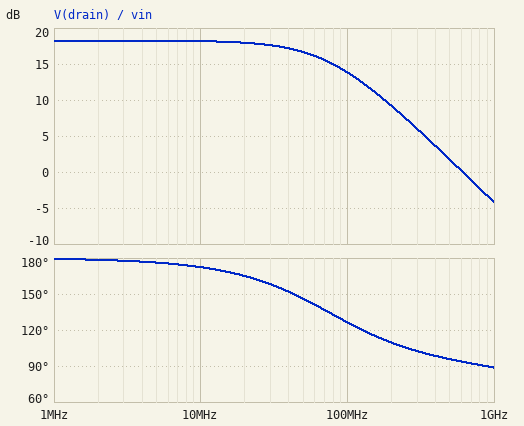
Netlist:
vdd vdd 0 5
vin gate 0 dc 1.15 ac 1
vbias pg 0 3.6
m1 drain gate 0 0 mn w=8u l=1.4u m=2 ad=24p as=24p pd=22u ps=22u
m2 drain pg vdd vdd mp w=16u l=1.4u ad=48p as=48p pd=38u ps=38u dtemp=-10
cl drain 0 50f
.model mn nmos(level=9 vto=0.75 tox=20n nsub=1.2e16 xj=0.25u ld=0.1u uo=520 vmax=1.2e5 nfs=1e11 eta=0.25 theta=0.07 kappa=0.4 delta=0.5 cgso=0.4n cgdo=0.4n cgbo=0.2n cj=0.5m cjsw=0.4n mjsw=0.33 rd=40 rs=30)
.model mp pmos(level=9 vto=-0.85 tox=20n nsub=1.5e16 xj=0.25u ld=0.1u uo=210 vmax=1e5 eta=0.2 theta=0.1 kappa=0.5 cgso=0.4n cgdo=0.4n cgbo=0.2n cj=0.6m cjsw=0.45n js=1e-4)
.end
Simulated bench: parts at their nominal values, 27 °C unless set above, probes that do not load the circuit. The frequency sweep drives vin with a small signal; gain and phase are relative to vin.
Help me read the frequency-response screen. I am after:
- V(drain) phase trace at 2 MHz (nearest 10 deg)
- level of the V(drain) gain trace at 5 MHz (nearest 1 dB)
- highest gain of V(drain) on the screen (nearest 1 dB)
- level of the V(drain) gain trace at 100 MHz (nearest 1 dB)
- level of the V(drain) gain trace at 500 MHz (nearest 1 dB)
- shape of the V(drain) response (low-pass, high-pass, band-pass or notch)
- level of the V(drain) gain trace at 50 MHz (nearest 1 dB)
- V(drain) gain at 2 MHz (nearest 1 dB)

180 deg
18 dB
18 dB
14 dB
2 dB
low-pass
17 dB
18 dB
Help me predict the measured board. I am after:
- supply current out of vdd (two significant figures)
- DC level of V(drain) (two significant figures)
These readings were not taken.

130 µA
1.2 V
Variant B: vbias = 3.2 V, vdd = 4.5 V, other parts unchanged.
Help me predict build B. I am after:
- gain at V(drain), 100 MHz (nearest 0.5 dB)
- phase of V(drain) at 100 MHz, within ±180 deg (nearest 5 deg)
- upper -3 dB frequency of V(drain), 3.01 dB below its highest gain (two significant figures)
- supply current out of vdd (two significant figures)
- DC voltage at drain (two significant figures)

13.0 dB
120 deg
64 MHz
100 µA
450 mV
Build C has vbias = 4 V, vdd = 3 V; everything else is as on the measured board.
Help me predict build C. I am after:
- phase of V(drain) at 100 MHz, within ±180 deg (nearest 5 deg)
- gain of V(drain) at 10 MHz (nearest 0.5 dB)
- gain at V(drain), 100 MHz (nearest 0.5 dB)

80 deg
-51.0 dB
-31.0 dB
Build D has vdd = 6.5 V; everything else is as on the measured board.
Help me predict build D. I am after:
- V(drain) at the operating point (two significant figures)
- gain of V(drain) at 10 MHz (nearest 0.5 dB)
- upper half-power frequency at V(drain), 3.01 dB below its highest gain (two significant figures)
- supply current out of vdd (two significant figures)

6.0 V
1.5 dB
750 MHz
380 µA
